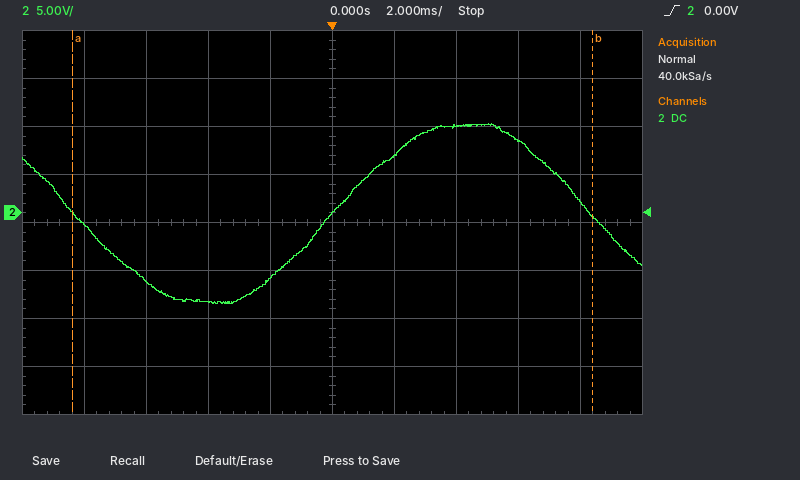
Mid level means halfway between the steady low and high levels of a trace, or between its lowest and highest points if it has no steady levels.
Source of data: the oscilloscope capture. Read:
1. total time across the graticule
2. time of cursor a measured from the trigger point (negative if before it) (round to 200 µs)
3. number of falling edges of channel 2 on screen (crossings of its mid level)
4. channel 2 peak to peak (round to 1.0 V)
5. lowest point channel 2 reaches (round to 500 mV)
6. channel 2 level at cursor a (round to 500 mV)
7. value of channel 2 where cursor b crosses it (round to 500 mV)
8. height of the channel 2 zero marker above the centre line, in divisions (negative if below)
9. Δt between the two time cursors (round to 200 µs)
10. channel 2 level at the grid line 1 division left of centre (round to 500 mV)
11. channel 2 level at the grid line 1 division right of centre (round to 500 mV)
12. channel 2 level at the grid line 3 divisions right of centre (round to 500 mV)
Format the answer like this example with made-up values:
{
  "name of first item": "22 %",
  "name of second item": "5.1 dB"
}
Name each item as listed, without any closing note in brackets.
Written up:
{
  "total time across the graticule": "20 ms",
  "time of cursor a measured from the trigger point (negative if before it)": "-8.4 ms",
  "number of falling edges of channel 2 on screen": "2",
  "channel 2 peak to peak": "19.0 V",
  "lowest point channel 2 reaches": "-9.5 V",
  "channel 2 level at cursor a": "0.0 V",
  "value of channel 2 where cursor b crosses it": "-500 mV",
  "height of the channel 2 zero marker above the centre line, in divisions": "+0.2 div",
  "Δt between the two time cursors": "16.8 ms",
  "channel 2 level at the grid line 1 division left of centre": "-7.0 V",
  "channel 2 level at the grid line 1 division right of centre": "6.0 V",
  "channel 2 level at the grid line 3 divisions right of centre": "7.5 V"
}
